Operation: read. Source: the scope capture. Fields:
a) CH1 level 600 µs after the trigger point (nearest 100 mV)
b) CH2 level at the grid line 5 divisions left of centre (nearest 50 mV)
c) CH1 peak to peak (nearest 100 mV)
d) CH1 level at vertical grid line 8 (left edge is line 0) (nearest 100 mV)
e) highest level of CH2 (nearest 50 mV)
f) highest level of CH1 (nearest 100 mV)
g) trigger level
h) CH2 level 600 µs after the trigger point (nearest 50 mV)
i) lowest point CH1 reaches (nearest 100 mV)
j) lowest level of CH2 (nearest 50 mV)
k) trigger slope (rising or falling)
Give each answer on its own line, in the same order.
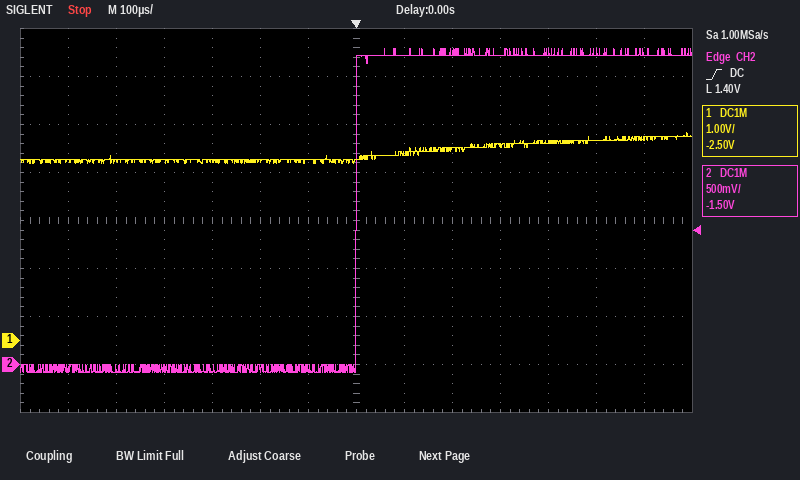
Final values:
4.2 V
-50 mV
600 mV
3.9 V
3.30 V
4.3 V
1.40 V
3.25 V
3.7 V
-100 mV
rising
